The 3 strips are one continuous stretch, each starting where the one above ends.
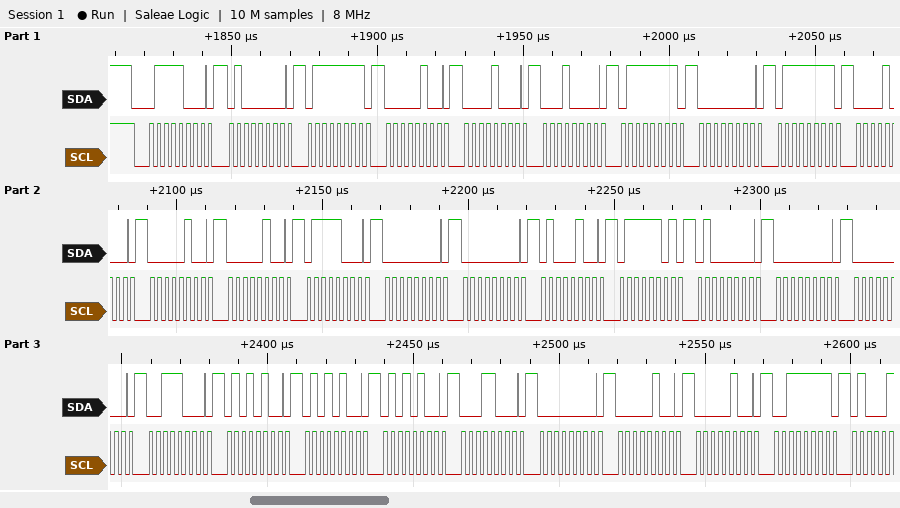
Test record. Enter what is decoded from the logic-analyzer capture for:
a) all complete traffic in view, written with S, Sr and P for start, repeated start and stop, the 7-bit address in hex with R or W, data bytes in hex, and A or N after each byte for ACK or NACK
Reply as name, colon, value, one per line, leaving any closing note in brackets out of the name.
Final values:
all complete traffic in view, written with S, Sr and P for start, repeated start and stop, the 7-bit address in hex with R or W, data bytes in hex, and A or N after each byte for ACK or NACK: S 3CW A 40 A 7F A 04 A 08 A 10 A 7F A 00 A 7F A 08 A 04 A 04 A 78 A 00 A 00 A 44 A 7D A 40 A 00 A 00 A 38 A 54 A 54 A 54 A 18 A 00 A 04 A 04 A 3F A
